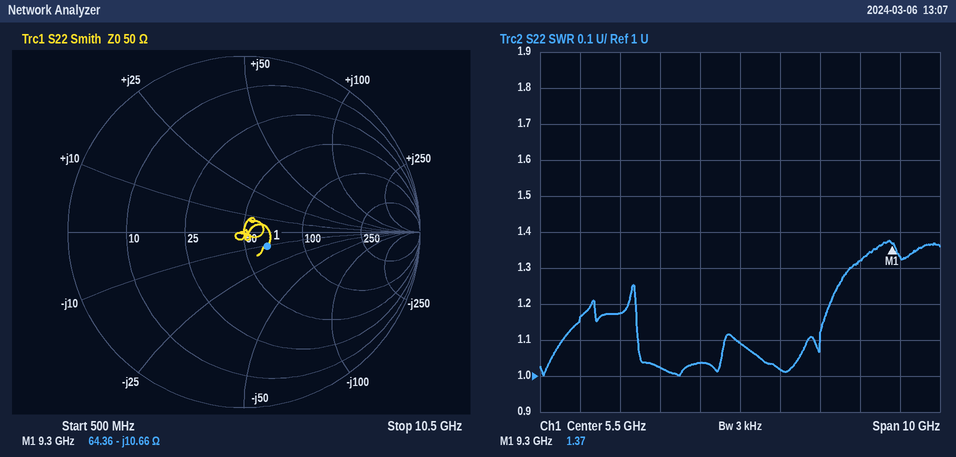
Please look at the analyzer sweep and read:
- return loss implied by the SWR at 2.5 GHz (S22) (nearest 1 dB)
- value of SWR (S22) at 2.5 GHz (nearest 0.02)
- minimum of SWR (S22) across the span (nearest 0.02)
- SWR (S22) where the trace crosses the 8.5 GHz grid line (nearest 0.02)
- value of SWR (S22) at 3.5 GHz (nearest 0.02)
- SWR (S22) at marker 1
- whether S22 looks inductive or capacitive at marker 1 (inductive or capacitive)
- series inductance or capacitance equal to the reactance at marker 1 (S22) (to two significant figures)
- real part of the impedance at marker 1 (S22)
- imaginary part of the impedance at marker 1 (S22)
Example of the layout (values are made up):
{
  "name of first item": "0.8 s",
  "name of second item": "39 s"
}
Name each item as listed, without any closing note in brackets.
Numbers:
{
  "return loss implied by the SWR at 2.5 GHz (S22)": "22 dB",
  "value of SWR (S22) at 2.5 GHz": "1.18",
  "minimum of SWR (S22) across the span": "1.00",
  "SWR (S22) where the trace crosses the 8.5 GHz grid line": "1.32",
  "value of SWR (S22) at 3.5 GHz": "1.02",
  "SWR (S22) at marker 1": "1.37",
  "whether S22 looks inductive or capacitive at marker 1": "capacitive",
  "series inductance or capacitance equal to the reactance at marker 1 (S22)": "1.6 pF",
  "real part of the impedance at marker 1": "64.36 Ω",
  "imaginary part of the impedance at marker 1": "-10.66 Ω"
}
